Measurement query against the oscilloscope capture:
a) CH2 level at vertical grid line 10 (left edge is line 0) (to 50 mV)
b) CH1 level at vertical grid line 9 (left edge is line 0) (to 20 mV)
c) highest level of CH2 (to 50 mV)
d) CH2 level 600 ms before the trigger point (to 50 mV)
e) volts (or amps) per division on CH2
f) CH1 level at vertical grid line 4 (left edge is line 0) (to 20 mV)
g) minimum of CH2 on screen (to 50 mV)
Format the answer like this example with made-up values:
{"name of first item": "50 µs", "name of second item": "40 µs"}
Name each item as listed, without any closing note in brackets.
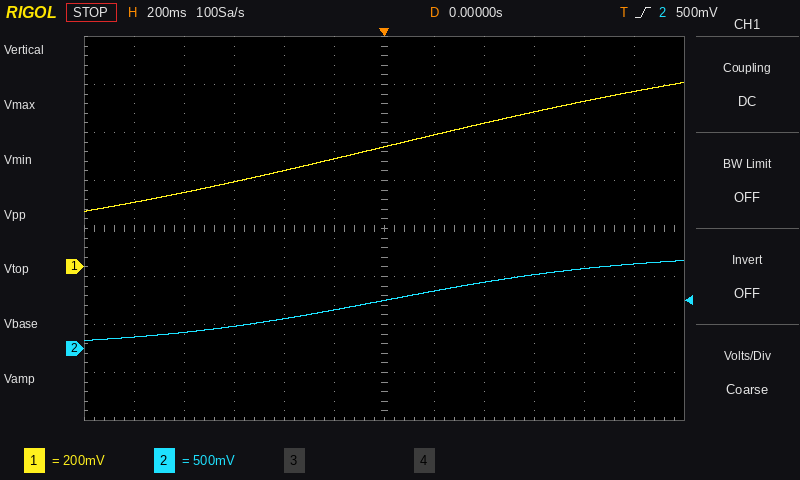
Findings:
{"CH2 level at vertical grid line 10 (left edge is line 0)": "850 mV", "CH1 level at vertical grid line 9 (left edge is line 0)": "640 mV", "highest level of CH2": "900 mV", "CH2 level 600 ms before the trigger point": "250 mV", "volts (or amps) per division on CH2": "500 mV", "CH1 level at vertical grid line 4 (left edge is line 0)": "400 mV", "minimum of CH2 on screen": "100 mV"}
